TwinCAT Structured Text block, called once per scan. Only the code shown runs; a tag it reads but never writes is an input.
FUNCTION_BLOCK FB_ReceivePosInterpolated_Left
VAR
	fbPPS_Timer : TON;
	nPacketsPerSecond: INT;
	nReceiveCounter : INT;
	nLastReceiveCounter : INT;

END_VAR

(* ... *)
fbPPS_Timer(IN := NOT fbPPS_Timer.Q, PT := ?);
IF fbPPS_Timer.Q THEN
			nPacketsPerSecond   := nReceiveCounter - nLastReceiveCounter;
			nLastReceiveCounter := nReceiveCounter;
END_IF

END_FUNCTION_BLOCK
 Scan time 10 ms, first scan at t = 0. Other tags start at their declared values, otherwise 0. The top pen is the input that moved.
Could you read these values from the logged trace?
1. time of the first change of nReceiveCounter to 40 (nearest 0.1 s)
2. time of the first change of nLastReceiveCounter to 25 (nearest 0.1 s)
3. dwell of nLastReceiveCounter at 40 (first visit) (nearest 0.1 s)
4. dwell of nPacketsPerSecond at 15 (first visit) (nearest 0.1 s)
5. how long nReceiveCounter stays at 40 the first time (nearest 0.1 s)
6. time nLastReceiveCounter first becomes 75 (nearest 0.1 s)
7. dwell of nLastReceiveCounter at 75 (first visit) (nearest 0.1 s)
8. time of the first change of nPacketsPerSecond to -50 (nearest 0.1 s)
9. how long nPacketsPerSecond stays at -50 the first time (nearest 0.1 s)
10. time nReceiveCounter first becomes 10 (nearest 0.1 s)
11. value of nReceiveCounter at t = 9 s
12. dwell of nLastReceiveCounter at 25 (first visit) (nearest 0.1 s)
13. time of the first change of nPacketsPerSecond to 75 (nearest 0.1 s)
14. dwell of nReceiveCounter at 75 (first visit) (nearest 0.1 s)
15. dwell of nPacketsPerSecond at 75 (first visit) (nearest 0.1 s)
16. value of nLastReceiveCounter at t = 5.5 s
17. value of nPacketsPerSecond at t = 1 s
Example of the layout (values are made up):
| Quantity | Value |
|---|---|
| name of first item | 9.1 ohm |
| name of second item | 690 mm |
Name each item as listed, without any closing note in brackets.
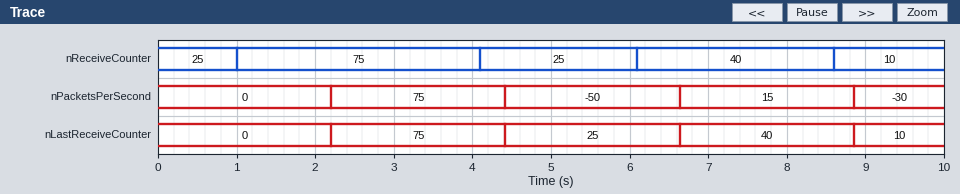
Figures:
| Quantity | Value |
|---|---|
| time of the first change of nReceiveCounter to 40 | 6.1 s |
| time of the first change of nLastReceiveCounter to 25 | 4.4 s |
| dwell of nLastReceiveCounter at 40 (first visit) | 2.2 s |
| dwell of nPacketsPerSecond at 15 (first visit) | 2.2 s |
| how long nReceiveCounter stays at 40 the first time | 2.5 s |
| time nLastReceiveCounter first becomes 75 | 2.2 s |
| dwell of nLastReceiveCounter at 75 (first visit) | 2.2 s |
| time of the first change of nPacketsPerSecond to -50 | 4.4 s |
| how long nPacketsPerSecond stays at -50 the first time | 2.2 s |
| time nReceiveCounter first becomes 10 | 8.6 s |
| value of nReceiveCounter at t = 9 s | 10 |
| dwell of nLastReceiveCounter at 25 (first visit) | 2.2 s |
| time of the first change of nPacketsPerSecond to 75 | 2.2 s |
| dwell of nReceiveCounter at 75 (first visit) | 3.1 s |
| dwell of nPacketsPerSecond at 75 (first visit) | 2.2 s |
| value of nLastReceiveCounter at t = 5.5 s | 25 |
| value of nPacketsPerSecond at t = 1 s | 0 |
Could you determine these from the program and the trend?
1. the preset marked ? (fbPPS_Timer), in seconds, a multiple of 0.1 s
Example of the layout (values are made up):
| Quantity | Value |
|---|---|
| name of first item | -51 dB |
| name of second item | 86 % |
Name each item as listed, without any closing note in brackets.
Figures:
| Quantity | Value |
|---|---|
| the preset marked ? (fbPPS_Timer), in seconds, a multiple of 0.1 s | 2.2 s |
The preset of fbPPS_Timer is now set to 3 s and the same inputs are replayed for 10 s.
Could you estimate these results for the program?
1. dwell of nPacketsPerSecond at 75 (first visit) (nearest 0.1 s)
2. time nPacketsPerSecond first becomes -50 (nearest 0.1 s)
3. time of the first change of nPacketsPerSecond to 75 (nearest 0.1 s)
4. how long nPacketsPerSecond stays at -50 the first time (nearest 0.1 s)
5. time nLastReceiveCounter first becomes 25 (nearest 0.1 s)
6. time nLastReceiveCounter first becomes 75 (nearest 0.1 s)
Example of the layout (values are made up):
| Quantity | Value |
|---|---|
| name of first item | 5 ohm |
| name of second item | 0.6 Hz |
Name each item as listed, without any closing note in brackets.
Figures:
| Quantity | Value |
|---|---|
| dwell of nPacketsPerSecond at 75 (first visit) | 3.0 s |
| time nPacketsPerSecond first becomes -50 | 6.0 s |
| time of the first change of nPacketsPerSecond to 75 | 3.0 s |
| how long nPacketsPerSecond stays at -50 the first time | 3.0 s |
| time nLastReceiveCounter first becomes 25 | 6.0 s |
| time nLastReceiveCounter first becomes 75 | 3.0 s |
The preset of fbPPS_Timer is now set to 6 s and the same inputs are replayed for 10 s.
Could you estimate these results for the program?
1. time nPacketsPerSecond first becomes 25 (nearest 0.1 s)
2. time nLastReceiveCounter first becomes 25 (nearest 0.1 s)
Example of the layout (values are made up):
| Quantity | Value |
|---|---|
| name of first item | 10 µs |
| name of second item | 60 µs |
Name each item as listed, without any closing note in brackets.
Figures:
| Quantity | Value |
|---|---|
| time nPacketsPerSecond first becomes 25 | 6.0 s |
| time nLastReceiveCounter first becomes 25 | 6.0 s |
